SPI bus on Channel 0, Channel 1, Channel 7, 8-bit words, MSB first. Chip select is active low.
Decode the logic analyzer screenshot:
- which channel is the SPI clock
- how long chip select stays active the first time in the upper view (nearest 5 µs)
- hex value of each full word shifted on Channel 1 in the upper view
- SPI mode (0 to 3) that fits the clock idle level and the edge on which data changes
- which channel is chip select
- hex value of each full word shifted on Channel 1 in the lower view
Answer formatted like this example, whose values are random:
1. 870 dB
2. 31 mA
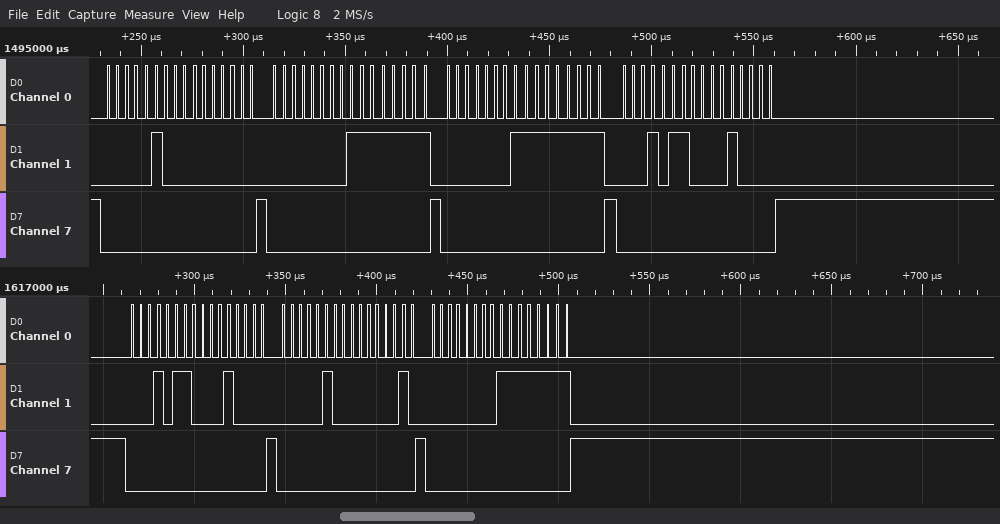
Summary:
1. Channel 0
2. 75 µs
3. 04, 00, 00, FF, 01, FF, 16, 10
4. 1
5. Channel 7
6. 16, 10, 04, 02, 00, FF
